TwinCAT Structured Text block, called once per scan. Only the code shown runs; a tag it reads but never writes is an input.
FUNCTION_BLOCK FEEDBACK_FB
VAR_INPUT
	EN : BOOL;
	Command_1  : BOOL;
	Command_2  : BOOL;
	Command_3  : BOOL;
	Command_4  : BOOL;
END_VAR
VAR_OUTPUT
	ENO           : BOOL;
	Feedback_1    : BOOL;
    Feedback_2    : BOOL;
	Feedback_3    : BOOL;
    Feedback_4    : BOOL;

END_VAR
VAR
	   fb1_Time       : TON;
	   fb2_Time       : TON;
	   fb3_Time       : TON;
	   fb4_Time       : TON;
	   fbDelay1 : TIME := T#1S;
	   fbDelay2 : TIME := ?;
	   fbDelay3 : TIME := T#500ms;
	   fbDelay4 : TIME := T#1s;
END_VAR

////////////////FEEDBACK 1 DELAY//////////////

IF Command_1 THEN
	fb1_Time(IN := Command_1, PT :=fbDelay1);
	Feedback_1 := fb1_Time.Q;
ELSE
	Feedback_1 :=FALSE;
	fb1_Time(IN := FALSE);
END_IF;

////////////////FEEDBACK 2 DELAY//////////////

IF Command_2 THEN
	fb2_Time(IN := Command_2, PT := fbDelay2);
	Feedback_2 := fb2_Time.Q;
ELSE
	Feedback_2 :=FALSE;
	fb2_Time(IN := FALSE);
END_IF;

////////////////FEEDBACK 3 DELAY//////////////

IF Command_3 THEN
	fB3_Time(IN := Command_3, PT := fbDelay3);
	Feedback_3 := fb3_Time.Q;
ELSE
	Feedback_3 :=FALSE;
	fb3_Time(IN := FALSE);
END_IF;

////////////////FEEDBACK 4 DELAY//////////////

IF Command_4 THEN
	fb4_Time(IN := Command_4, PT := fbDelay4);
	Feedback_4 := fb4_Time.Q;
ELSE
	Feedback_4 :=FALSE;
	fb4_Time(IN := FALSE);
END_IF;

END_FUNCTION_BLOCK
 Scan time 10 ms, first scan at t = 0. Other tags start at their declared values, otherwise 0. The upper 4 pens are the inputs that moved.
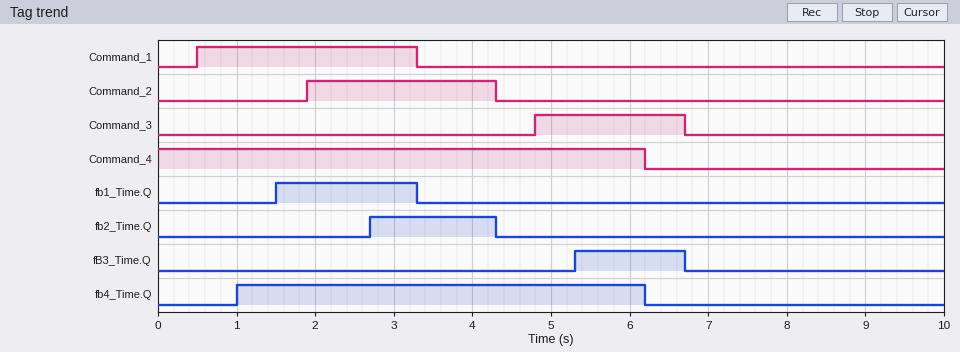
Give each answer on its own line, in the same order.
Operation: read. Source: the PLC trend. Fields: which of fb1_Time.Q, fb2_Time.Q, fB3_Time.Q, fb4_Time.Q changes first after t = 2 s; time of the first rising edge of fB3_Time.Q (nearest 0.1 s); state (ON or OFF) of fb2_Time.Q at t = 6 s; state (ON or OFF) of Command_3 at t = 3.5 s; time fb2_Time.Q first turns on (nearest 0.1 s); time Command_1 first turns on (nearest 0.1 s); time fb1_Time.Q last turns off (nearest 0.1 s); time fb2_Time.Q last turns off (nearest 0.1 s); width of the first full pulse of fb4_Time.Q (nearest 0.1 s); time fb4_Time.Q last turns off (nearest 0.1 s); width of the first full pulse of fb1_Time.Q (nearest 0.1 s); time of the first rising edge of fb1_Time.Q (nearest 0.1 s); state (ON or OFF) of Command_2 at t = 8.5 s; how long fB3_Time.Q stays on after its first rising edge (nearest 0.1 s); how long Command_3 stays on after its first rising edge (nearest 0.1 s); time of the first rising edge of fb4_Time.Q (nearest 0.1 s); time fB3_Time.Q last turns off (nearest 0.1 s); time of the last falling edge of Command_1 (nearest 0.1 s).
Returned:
fb2_Time.Q
5.3 s
OFF
OFF
2.7 s
0.5 s
3.3 s
4.3 s
5.2 s
6.2 s
1.8 s
1.5 s
OFF
1.4 s
1.9 s
1.0 s
6.7 s
3.3 s
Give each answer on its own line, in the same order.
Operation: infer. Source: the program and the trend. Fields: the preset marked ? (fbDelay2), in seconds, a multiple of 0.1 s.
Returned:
0.8 s
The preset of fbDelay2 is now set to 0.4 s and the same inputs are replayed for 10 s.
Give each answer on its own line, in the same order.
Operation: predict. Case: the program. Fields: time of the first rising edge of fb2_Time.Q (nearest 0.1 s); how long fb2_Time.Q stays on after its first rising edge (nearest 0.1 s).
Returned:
2.3 s
2.0 s
